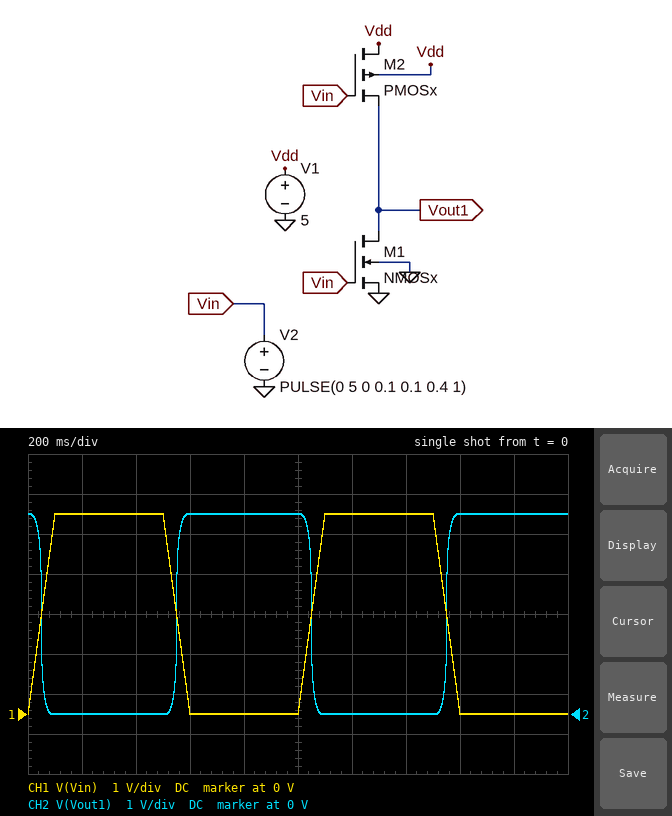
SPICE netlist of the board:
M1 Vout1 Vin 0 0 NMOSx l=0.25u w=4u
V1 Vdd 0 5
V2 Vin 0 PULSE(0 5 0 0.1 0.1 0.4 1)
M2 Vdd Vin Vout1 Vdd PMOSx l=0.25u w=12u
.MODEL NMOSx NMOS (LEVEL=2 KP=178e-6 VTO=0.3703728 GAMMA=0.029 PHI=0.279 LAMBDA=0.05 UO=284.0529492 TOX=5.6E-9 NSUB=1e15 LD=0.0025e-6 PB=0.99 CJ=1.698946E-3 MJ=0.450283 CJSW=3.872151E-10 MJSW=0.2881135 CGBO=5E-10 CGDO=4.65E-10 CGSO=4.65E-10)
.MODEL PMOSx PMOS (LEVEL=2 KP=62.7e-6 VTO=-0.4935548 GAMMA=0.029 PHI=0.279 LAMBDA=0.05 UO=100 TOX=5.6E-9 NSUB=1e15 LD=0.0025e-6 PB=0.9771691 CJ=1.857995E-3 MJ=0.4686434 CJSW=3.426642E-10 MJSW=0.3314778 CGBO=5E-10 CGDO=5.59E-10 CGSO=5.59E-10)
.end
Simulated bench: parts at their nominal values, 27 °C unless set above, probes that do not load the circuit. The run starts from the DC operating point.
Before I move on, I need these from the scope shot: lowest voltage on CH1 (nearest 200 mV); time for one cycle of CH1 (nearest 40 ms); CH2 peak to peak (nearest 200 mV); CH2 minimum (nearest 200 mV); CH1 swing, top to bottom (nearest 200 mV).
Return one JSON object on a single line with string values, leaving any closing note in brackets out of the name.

{"lowest voltage on CH1": "0 V", "time for one cycle of CH1": "1.00 s", "CH2 peak to peak": "5.0 V", "CH2 minimum": "0 V", "CH1 swing, top to bottom": "5.0 V"}
